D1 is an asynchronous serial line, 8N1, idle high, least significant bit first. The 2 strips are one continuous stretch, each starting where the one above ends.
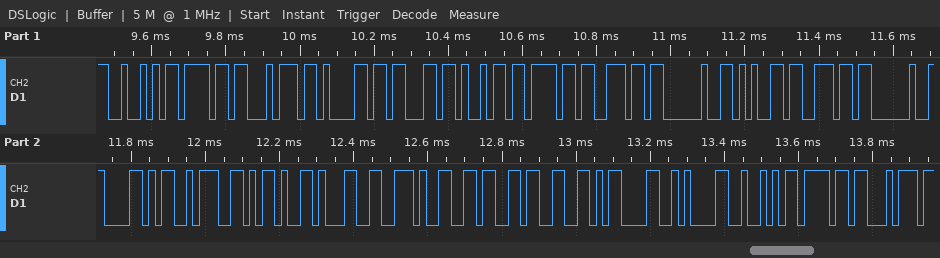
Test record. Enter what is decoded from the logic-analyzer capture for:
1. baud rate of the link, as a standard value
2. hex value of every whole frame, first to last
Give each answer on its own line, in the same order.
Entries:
57600 baud
52 6F 74 61 63 69 6F 6E 20 65 6E 20 58 3A 2D 31 2E 36 33 0D 0A 52 6F 74
